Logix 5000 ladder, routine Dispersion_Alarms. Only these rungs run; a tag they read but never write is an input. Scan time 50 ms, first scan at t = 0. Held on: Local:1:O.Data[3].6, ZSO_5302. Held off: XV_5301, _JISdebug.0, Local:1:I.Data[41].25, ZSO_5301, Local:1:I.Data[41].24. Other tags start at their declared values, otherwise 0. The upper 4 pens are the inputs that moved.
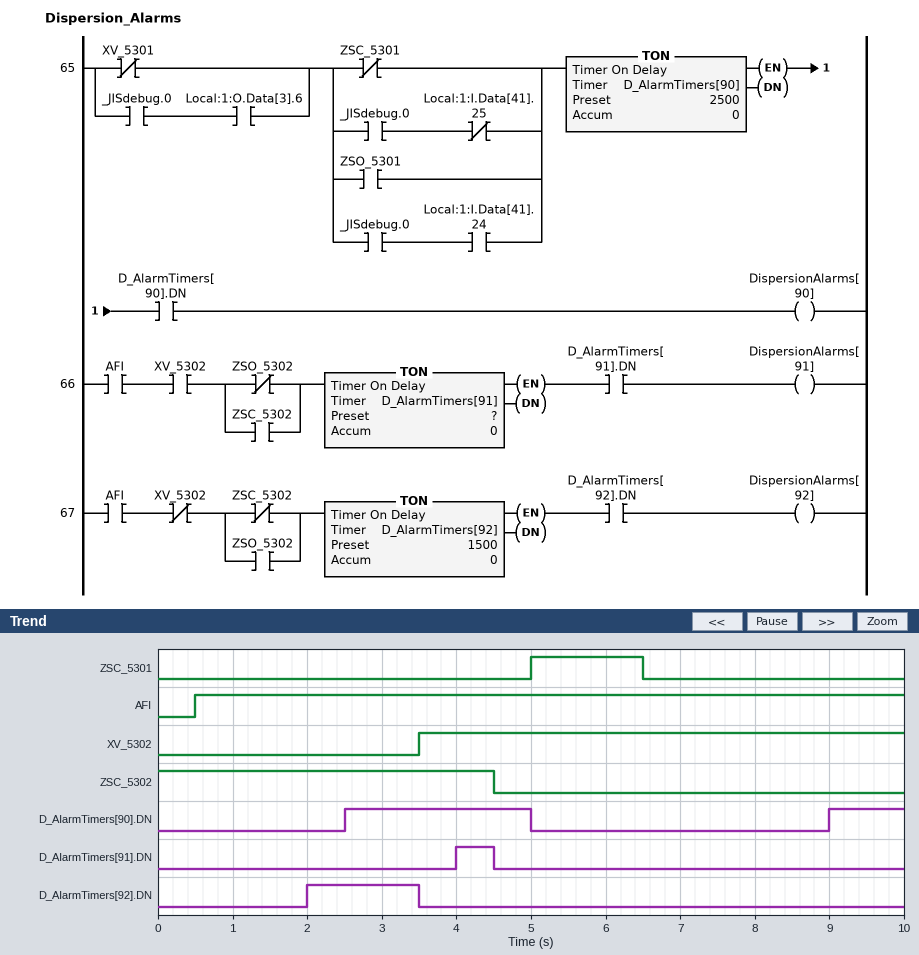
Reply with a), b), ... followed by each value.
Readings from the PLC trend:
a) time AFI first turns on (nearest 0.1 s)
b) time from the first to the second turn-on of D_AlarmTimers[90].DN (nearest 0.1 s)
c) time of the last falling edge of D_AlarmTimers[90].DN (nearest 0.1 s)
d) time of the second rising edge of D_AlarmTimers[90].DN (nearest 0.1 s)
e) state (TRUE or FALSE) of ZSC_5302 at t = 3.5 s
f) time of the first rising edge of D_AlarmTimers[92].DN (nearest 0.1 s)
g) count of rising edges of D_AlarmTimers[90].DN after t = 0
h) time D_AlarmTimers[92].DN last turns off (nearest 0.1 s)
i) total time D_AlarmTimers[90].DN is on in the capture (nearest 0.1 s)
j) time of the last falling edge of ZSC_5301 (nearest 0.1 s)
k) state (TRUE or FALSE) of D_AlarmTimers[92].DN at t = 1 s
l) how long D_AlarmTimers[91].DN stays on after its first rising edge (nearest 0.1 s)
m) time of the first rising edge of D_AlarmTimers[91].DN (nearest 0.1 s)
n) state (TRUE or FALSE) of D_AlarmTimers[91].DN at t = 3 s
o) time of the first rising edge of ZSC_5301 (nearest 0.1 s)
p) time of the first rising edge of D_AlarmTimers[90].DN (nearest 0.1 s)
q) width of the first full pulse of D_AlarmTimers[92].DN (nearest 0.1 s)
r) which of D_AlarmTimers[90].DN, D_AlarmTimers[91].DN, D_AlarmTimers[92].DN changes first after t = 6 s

a) 0.5 s
b) 6.5 s
c) 5.0 s
d) 9.0 s
e) TRUE
f) 2.0 s
g) 2
h) 3.5 s
i) 3.5 s
j) 6.5 s
k) FALSE
l) 0.5 s
m) 4.0 s
n) FALSE
o) 5.0 s
p) 2.5 s
q) 1.5 s
r) D_AlarmTimers[90].DN
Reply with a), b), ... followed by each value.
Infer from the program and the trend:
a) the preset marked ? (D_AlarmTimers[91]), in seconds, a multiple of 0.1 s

a) 0.5 s
